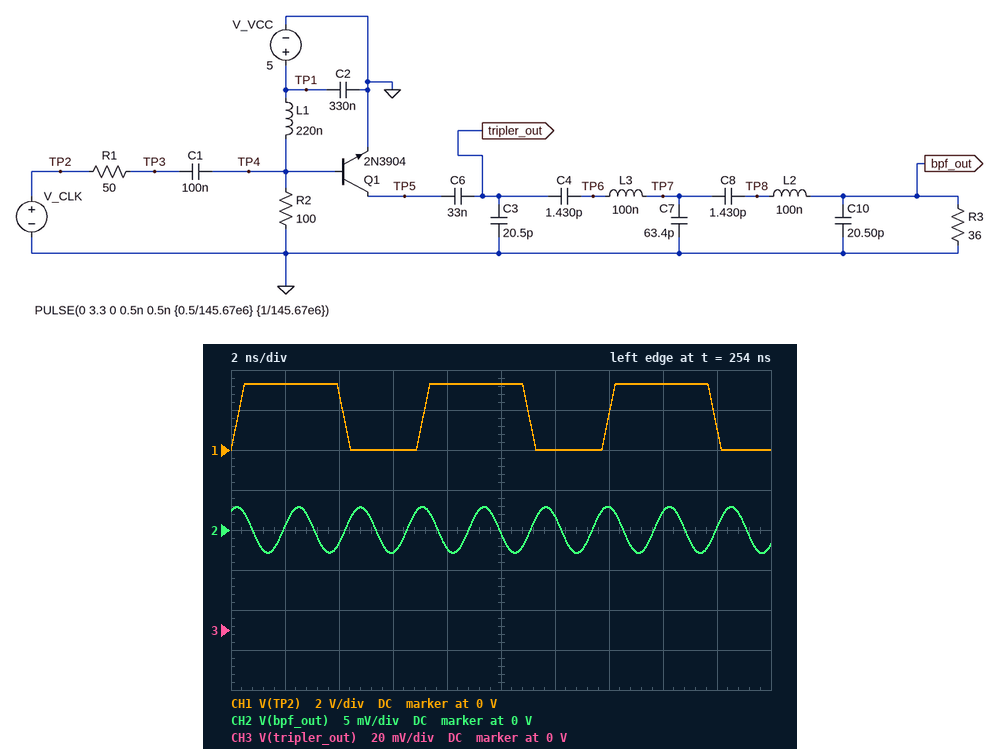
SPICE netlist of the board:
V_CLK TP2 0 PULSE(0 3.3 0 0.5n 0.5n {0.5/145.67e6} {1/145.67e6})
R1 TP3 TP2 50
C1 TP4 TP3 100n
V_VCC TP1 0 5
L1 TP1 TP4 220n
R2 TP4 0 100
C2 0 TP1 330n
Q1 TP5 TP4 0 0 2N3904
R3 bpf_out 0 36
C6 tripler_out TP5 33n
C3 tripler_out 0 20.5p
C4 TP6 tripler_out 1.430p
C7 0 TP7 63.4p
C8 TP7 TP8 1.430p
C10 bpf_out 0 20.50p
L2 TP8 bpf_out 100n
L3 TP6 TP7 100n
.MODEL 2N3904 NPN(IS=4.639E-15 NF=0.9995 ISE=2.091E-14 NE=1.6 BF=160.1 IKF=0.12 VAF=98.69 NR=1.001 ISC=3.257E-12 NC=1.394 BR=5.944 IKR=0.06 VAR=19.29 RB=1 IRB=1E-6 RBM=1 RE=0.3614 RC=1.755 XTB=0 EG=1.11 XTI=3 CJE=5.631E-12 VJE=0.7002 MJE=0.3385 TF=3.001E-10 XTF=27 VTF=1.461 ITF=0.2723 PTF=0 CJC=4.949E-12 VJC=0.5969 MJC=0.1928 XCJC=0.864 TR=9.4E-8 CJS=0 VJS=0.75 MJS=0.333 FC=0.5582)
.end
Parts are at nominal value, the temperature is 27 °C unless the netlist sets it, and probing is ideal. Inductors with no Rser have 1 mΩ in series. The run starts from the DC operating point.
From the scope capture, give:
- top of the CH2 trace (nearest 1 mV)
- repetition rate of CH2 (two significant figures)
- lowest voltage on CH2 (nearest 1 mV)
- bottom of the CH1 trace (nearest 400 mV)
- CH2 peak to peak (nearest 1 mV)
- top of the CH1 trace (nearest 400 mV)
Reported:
3 mV
440 MHz
-3 mV
0 V
6 mV
3.2 V
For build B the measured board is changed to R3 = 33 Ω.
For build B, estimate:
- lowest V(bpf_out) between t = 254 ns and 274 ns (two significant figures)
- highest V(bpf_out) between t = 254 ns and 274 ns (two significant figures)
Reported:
-2.8 mV
2.8 mV
